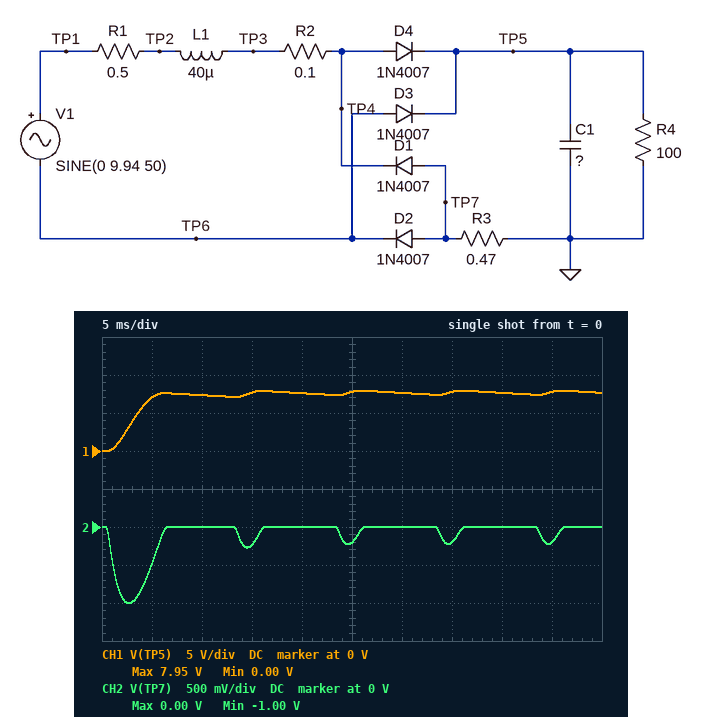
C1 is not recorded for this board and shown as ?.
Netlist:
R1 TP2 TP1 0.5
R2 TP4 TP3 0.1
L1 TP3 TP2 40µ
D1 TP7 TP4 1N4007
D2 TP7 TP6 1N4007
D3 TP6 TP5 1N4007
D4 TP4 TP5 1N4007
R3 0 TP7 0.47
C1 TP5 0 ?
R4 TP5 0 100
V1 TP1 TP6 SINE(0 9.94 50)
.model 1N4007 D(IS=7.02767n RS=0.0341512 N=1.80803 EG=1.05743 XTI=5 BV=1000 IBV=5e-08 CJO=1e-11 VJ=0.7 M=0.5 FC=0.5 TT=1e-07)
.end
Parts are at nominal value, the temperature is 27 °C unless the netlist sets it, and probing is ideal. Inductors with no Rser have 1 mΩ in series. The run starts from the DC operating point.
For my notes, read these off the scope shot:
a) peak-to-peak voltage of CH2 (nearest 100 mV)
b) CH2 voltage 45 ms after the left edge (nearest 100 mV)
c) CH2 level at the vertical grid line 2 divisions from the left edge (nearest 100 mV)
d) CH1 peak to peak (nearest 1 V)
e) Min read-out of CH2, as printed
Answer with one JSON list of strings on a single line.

["1.0 V", "-200 mV", "0 V", "8 V", "-1.00 V"]
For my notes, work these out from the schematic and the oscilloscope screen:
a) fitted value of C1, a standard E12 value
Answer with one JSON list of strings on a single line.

["1 mF"]
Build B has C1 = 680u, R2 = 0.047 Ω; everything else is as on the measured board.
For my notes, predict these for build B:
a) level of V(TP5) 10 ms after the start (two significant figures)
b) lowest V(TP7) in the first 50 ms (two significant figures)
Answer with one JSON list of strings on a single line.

["7.5 V", "-770 mV"]
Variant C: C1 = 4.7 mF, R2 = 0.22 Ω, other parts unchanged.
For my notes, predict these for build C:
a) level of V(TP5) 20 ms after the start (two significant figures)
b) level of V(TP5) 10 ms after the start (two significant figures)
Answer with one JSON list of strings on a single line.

["5.9 V", "4.4 V"]
